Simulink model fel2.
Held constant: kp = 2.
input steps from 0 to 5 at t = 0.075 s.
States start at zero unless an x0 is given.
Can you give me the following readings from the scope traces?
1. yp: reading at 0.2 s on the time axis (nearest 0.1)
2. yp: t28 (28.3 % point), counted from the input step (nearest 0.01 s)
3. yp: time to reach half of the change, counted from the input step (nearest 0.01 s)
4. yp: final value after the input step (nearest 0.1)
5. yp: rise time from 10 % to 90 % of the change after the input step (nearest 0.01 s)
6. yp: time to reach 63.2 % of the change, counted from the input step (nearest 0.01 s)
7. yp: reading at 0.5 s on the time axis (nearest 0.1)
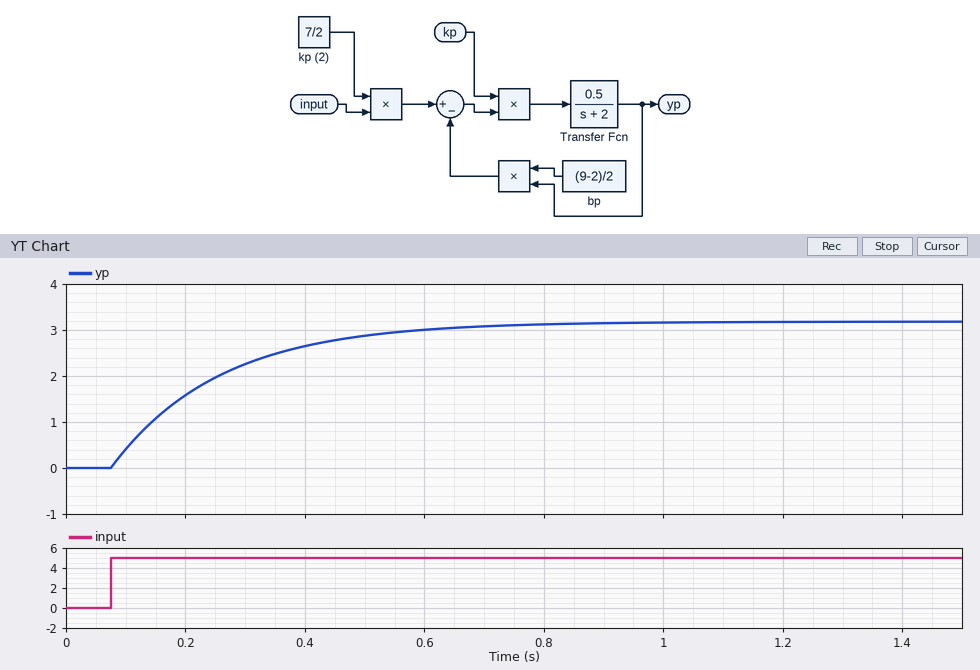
1.6
0.06 s
0.13 s
3.2
0.40 s
0.18 s
2.9
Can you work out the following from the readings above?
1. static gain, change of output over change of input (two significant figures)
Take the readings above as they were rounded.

0.64
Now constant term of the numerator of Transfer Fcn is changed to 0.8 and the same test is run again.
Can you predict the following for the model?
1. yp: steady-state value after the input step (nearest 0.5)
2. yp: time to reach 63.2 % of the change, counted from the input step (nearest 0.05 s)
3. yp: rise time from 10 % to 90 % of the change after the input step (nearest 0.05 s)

3.5
0.15 s
0.30 s
